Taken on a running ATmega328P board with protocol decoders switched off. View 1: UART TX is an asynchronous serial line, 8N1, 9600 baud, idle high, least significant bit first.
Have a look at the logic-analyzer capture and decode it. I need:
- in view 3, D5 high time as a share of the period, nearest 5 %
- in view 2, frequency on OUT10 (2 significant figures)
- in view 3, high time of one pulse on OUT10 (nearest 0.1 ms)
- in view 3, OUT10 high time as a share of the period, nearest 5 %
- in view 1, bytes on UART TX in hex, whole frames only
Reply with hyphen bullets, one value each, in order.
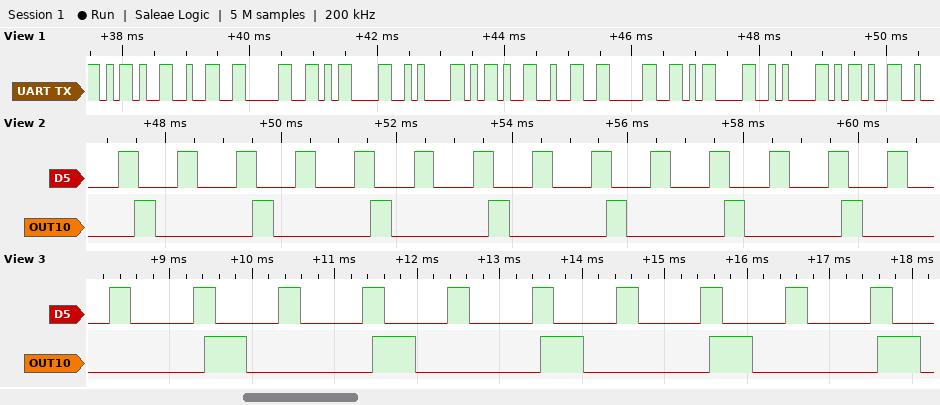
- 25 %
- 490 Hz
- 0.5 ms
- 25 %
- 2D 32 30 0D 0A 2D 32 30 0D 0A 2D
